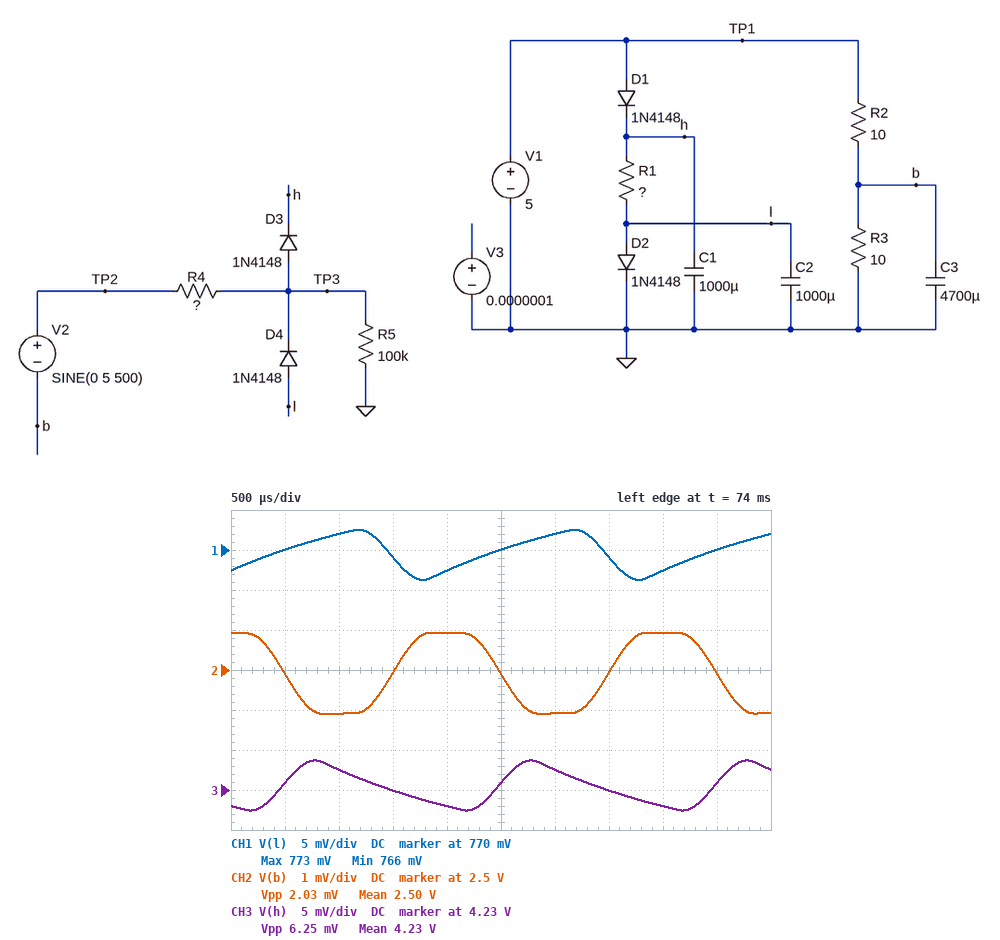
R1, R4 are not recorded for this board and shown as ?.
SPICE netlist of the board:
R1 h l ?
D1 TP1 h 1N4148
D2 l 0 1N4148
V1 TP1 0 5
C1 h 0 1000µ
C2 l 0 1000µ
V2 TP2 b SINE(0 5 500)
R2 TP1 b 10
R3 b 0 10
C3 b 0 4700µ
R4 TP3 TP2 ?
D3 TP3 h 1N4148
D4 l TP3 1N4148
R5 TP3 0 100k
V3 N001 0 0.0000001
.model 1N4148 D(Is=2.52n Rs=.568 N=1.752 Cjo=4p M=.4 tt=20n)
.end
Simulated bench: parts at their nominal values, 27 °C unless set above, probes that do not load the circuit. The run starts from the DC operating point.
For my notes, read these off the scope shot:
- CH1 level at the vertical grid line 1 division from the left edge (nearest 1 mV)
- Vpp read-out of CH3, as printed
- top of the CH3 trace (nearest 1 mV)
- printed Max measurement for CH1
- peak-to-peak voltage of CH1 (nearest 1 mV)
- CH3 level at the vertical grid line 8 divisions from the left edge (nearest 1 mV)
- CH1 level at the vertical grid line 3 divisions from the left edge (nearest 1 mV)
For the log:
770 mV
6.25 mV
4.234 V
773 mV
6 mV
4.228 V
769 mV
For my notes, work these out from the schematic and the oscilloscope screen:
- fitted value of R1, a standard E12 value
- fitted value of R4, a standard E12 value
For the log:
82 Ω
120 Ω
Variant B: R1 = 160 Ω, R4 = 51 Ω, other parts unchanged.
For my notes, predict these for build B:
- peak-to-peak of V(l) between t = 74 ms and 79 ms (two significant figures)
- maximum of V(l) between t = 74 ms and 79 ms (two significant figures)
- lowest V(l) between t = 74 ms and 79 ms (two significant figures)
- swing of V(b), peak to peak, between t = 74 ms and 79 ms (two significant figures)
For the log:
14 mV
710 mV
700 mV
4.5 mV
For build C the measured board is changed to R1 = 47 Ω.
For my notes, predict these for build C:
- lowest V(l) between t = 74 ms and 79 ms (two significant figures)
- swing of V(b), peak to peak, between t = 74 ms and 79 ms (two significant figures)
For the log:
810 mV
2.1 mV
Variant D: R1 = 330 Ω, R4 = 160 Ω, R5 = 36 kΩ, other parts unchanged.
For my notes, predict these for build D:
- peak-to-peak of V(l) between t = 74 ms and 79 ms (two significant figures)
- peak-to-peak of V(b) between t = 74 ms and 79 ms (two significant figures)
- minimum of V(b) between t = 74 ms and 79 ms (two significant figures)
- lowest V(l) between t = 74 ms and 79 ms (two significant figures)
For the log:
4.6 mV
1.5 mV
2.5 V
680 mV
